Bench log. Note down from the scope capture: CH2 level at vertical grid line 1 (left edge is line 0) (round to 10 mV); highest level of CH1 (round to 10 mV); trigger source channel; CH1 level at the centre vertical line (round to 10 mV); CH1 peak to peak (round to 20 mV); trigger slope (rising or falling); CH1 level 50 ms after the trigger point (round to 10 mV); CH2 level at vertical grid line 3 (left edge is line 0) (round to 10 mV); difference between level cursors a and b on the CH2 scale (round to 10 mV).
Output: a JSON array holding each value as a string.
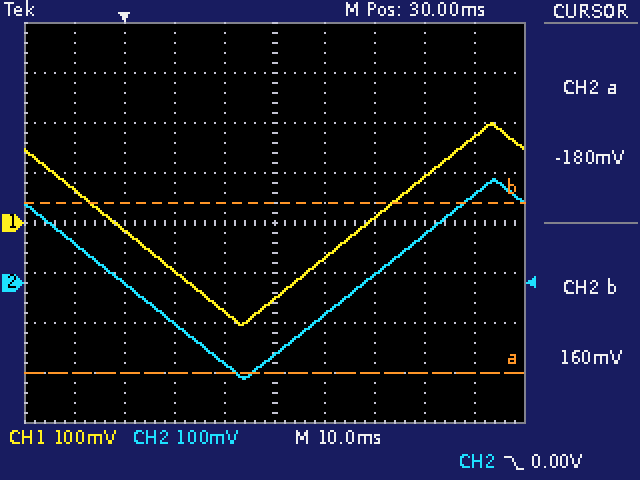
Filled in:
["80 mV", "200 mV", "CH2", "-150 mV", "400 mV", "falling", "10 mV", "-80 mV", "340 mV"]
